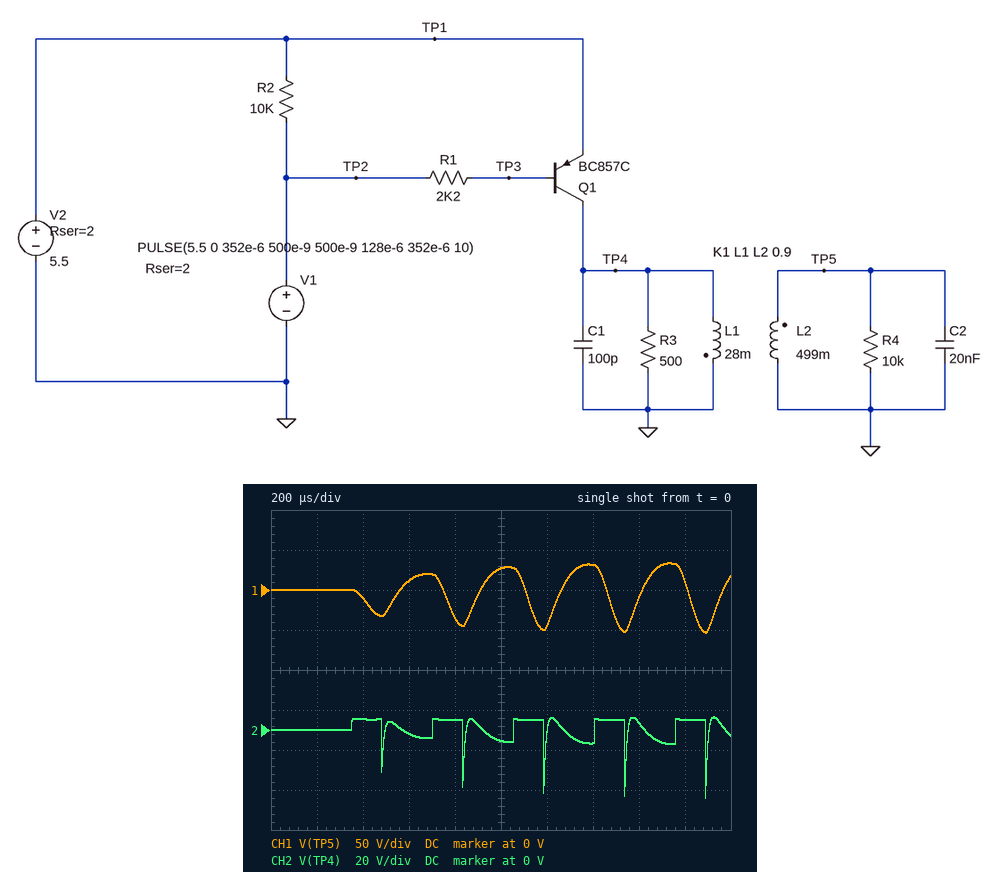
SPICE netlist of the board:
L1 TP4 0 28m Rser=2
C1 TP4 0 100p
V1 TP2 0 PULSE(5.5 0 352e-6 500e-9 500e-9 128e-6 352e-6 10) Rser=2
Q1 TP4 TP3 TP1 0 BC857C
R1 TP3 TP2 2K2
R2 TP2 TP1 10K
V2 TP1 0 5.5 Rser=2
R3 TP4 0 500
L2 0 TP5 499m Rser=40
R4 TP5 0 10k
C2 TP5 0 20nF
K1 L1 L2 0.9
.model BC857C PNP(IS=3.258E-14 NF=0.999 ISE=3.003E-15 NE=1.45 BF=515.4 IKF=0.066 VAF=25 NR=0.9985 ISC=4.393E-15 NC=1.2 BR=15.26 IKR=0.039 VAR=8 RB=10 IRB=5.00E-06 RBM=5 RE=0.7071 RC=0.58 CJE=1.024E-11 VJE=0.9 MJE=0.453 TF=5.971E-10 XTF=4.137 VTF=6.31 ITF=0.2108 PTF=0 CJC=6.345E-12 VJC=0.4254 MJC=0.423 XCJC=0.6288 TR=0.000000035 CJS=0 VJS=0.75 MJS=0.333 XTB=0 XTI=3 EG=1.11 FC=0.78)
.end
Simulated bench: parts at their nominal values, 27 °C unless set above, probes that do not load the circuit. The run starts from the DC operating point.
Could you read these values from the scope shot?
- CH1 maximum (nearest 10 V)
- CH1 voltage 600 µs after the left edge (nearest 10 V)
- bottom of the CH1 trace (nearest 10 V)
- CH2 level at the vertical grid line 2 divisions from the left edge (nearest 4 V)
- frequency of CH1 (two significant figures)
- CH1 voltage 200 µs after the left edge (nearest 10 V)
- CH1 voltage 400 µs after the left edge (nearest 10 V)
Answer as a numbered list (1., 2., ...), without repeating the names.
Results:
1. 30 V
2. 10 V
3. -50 V
4. 4 V
5. 2.8 kHz
6. 0 V
7. -10 V
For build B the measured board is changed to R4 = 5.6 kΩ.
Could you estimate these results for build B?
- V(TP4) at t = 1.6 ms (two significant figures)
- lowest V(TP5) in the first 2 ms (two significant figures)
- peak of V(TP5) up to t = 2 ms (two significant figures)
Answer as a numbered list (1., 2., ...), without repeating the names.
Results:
1. 1.5 V
2. -39 V
3. 23 V
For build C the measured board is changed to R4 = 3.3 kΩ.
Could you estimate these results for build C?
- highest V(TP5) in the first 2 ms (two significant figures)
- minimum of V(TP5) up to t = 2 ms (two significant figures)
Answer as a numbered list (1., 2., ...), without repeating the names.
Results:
1. 15 V
2. -29 V
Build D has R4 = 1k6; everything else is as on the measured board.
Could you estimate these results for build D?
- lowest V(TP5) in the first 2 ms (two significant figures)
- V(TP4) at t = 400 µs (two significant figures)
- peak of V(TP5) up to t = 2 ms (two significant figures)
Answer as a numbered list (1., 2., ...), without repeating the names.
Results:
1. -19 V
2. 5.3 V
3. 8.2 V
